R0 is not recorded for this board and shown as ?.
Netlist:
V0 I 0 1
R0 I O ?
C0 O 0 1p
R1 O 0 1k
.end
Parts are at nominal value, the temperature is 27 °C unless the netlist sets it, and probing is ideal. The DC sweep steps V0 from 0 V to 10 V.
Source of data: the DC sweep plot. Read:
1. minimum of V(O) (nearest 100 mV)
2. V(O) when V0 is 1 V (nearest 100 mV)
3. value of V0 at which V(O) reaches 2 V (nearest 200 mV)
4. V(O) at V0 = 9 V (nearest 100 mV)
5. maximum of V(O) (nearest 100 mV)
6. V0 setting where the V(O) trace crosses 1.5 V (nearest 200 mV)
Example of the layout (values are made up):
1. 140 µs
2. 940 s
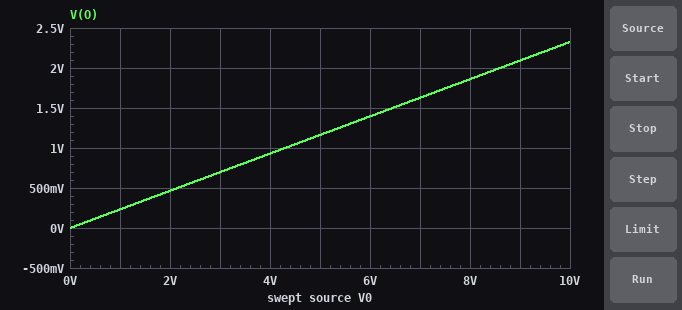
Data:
1. 0 V
2. 200 mV
3. 8.6 V
4. 2.1 V
5. 2.3 V
6. 6.4 V
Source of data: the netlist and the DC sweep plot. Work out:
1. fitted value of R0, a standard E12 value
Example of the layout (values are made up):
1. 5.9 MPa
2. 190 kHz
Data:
1. 3.3 kΩ
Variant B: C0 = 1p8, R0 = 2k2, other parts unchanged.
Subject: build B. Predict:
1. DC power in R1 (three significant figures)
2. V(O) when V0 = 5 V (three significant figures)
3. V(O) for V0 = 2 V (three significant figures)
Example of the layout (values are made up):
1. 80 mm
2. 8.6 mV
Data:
1. 97.7 µW
2. 1.56 V
3. 625 mV
